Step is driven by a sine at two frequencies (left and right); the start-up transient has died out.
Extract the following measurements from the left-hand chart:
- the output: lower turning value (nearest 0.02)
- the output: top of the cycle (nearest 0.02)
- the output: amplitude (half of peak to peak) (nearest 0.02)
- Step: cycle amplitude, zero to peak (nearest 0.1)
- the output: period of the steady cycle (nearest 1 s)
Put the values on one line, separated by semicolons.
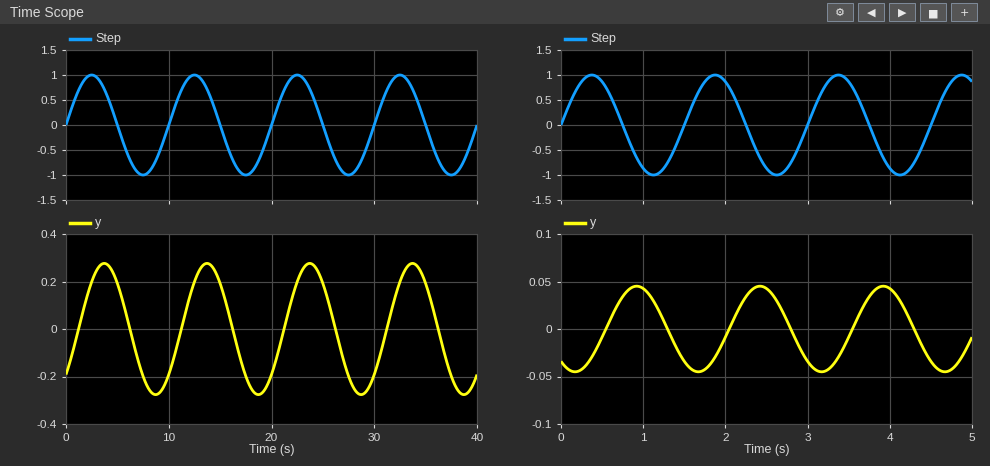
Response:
-0.28; 0.28; 0.28; 1.0; 10 s
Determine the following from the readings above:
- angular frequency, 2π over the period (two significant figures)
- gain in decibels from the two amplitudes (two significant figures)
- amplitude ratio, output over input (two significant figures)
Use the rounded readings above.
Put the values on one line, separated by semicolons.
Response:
0.63 rad/s; -11 dB; 0.28
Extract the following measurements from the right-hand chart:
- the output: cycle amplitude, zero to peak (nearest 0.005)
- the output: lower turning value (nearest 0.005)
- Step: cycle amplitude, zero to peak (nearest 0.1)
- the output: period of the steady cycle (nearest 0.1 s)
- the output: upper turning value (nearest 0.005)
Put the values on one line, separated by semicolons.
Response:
0.045; -0.045; 1.0; 1.5 s; 0.045
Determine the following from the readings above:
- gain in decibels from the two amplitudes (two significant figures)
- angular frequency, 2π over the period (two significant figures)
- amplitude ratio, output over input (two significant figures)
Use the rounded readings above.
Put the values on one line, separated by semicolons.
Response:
-27 dB; 4.2 rad/s; 0.045
